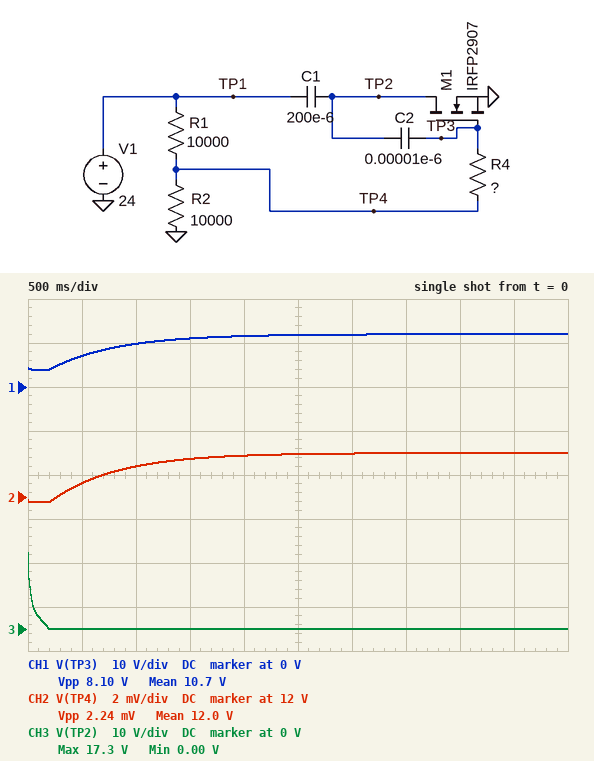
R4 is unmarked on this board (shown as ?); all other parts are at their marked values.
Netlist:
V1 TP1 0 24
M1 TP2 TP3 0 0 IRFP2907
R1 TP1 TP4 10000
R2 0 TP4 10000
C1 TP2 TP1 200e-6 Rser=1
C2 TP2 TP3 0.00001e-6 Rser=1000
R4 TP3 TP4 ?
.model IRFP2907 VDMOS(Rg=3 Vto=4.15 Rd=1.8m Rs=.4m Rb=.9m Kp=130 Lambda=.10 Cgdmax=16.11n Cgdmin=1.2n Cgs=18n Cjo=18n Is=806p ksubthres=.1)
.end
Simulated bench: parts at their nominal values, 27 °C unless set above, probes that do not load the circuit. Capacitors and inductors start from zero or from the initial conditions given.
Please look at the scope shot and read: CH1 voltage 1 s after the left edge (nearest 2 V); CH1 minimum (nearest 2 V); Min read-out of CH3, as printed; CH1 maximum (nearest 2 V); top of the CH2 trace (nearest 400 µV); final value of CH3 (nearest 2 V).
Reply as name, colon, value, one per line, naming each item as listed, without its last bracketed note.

CH1 voltage 1 s after the left edge: 10 V
CH1 minimum: 4 V
Min read-out of CH3, as printed: 0.00 V
CH1 maximum: 12 V
top of the CH2 trace: 12.0000 V
final value of CH3: 0 V
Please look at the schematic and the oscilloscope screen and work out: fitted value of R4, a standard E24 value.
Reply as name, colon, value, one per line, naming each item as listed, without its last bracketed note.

fitted value of R4, a standard E24 value: 18 MΩ
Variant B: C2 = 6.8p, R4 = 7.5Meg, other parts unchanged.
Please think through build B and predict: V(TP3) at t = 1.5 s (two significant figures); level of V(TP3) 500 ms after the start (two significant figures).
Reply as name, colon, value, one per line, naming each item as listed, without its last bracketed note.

V(TP3) at t = 1.5 s: 12 V
level of V(TP3) 500 ms after the start: 10 V
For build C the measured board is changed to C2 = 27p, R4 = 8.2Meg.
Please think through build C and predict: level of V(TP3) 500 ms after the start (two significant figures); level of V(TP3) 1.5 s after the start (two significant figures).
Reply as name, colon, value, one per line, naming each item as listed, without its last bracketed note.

level of V(TP3) 500 ms after the start: 10 V
level of V(TP3) 1.5 s after the start: 12 V
